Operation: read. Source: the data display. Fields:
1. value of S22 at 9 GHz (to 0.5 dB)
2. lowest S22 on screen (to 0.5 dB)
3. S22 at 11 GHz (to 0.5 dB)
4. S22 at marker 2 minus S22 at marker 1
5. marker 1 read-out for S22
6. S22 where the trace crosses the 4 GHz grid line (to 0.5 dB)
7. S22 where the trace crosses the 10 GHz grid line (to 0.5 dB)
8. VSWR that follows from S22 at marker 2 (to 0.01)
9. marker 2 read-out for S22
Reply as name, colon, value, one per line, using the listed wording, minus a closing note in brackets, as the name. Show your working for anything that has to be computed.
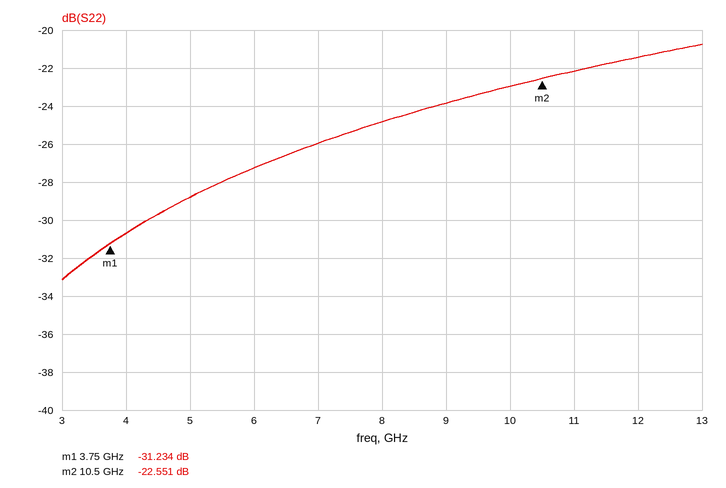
value of S22 at 9 GHz: -24.0 dB
lowest S22 on screen: -33.0 dB
S22 at 11 GHz: -22.0 dB
S22 at marker 2 minus S22 at marker 1: -22.551 − (-31.234) = 8.683 dB
marker 1 read-out for S22: -31.234 dB
S22 where the trace crosses the 4 GHz grid line: -30.5 dB
S22 where the trace crosses the 10 GHz grid line: -23.0 dB
VSWR that follows from S22 at marker 2: (1 + 0.0746)/(1 − 0.0746) ≈ 1.16
marker 2 read-out for S22: -22.551 dB
